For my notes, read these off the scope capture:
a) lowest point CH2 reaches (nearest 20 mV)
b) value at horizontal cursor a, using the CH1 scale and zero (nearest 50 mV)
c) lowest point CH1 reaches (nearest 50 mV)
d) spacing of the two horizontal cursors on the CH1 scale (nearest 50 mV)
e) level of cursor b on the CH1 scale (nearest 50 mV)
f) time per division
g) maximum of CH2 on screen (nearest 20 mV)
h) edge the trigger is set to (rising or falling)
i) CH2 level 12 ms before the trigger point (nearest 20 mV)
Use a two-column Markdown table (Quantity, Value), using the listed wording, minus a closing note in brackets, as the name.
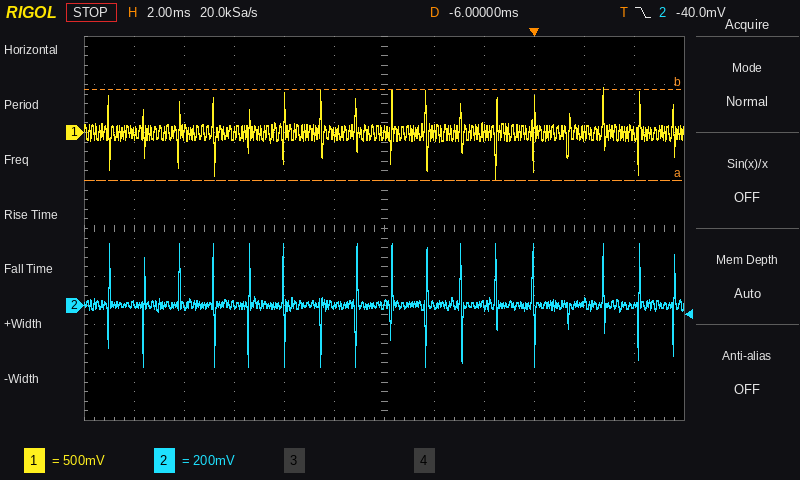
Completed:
| Quantity | Value |
|---|---|
| lowest point CH2 reaches | -260 mV |
| value at horizontal cursor a, using the CH1 scale and zero | -500 mV |
| lowest point CH1 reaches | -500 mV |
| spacing of the two horizontal cursors on the CH1 scale | 950 mV |
| level of cursor b on the CH1 scale | 450 mV |
| time per division | 2 ms |
| maximum of CH2 on screen | 260 mV |
| edge the trigger is set to | falling |
| CH2 level 12 ms before the trigger point | 0 mV |
